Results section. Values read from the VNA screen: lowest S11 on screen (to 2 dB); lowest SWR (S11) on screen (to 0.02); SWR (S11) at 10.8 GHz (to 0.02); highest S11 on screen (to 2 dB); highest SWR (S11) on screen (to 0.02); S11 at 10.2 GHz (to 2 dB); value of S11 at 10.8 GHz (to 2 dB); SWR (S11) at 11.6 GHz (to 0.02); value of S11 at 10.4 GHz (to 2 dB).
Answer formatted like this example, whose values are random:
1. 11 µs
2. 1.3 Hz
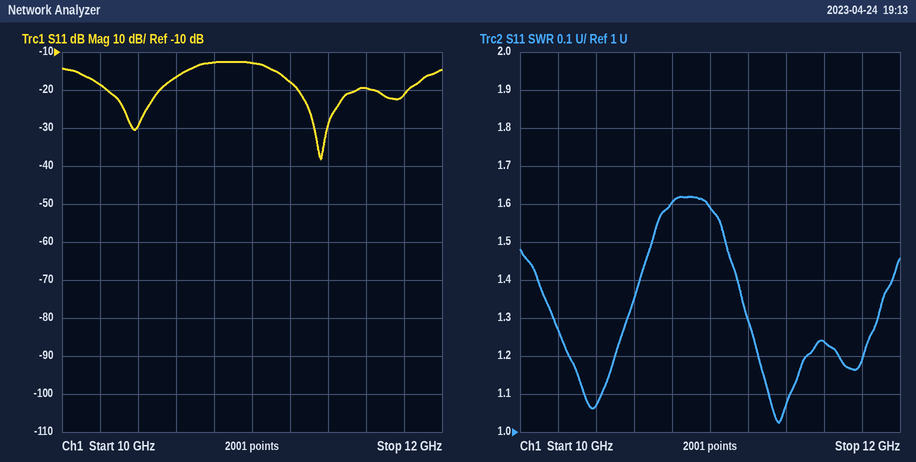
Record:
1. -38 dB
2. 1.02
3. 1.60
4. -12 dB
5. 1.62
6. -18 dB
7. -12 dB
8. 1.24
9. -30 dB
